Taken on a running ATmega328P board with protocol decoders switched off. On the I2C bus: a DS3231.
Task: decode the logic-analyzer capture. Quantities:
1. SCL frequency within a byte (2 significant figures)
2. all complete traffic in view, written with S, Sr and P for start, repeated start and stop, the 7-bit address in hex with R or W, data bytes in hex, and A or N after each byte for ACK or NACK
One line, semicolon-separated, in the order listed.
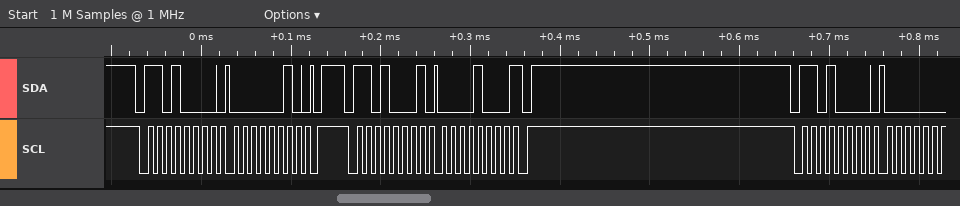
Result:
100 kHz; S 68W A 02 A P S 68R A 08 N P S 68W A
